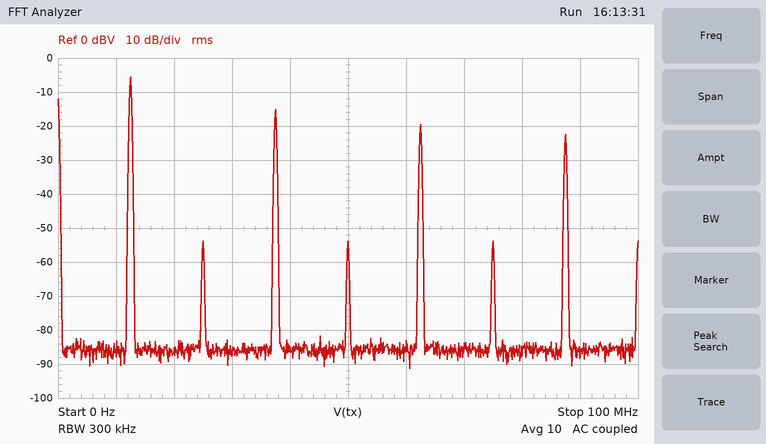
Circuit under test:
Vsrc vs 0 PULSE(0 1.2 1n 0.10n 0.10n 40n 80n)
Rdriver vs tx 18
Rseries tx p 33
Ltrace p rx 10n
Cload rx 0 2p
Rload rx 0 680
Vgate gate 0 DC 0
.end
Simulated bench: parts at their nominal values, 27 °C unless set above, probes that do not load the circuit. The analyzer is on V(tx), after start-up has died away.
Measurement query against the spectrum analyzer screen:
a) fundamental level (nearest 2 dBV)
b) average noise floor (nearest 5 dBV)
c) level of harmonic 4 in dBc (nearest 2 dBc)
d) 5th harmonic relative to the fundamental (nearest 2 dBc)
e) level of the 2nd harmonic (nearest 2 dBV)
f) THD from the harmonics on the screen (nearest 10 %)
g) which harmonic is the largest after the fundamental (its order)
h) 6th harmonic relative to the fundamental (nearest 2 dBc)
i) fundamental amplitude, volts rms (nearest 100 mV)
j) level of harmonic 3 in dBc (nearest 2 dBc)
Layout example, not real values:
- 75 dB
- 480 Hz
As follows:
- -6 dBV
- -85 dBV
- -48 dBc
- -14 dBc
- -54 dBV
- 40 %
- 3
- -48 dBc
- 500 mV
- -10 dBc
